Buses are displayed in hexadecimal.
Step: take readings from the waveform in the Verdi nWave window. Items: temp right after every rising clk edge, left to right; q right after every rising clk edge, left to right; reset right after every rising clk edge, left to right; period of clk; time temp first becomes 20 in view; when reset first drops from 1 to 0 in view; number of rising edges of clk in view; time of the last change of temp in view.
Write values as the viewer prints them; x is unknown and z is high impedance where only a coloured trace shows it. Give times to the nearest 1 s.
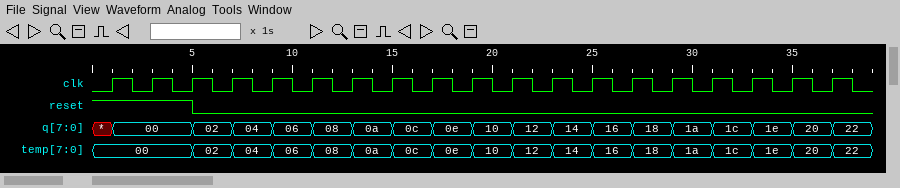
00, 00, 02, 04, 06, 08, 0a, 0c, 0e, 10, 12, 14, 16, 18, 1a, 1c, 1e, 20, 22
00, 00, 02, 04, 06, 08, 0a, 0c, 0e, 10, 12, 14, 16, 18, 1a, 1c, 1e, 20, 22
1 1 0 0 0 0 0 0 0 0 0 0 0 0 0 0 0 0 0
2 s
35 s
5 s
19
37 s
